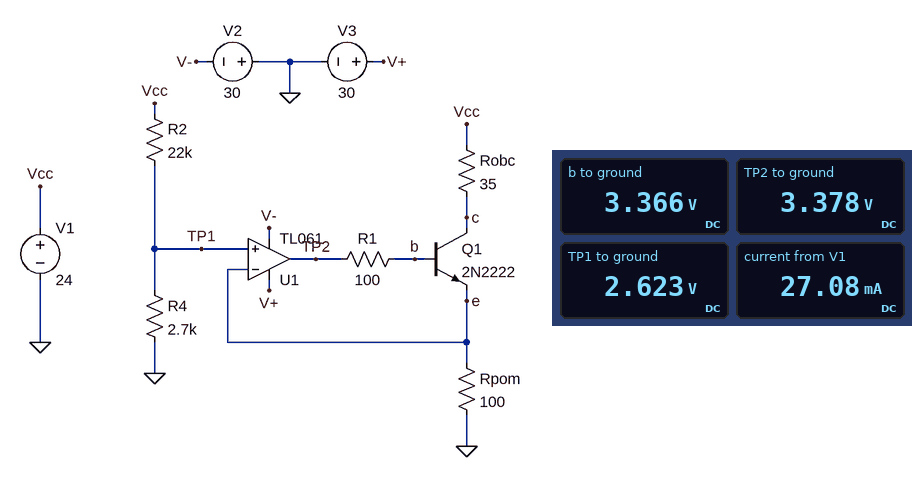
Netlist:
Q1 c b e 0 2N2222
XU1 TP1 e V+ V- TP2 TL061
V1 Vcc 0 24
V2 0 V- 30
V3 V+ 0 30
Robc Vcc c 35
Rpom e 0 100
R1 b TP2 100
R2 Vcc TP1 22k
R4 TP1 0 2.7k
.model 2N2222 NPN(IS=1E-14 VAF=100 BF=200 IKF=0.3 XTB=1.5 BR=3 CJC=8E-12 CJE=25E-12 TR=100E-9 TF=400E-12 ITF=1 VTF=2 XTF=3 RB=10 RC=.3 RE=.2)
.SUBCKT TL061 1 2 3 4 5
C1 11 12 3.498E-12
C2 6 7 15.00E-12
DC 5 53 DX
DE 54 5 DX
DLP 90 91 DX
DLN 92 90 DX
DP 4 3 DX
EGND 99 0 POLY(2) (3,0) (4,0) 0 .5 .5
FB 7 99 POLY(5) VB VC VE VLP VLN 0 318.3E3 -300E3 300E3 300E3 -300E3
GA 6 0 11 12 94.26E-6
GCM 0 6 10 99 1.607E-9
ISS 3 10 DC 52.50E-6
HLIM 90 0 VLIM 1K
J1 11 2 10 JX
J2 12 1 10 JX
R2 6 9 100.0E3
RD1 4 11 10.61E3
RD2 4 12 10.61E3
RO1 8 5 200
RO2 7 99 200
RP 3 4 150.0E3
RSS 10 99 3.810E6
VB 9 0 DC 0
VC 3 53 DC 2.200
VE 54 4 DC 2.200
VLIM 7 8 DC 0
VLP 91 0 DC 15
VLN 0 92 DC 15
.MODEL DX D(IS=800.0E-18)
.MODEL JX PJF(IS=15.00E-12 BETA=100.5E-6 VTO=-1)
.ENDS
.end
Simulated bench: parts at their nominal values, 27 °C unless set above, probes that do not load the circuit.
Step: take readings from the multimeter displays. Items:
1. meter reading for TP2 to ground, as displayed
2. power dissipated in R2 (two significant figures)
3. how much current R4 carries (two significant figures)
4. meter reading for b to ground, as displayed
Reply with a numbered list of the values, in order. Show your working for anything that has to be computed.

1. 3.378 V
2. (24 V - 2.623 V)^2 / 22 kΩ = 21 mW
3. (2.623 V) / 2.7 kΩ = 970 µA
4. 3.366 V
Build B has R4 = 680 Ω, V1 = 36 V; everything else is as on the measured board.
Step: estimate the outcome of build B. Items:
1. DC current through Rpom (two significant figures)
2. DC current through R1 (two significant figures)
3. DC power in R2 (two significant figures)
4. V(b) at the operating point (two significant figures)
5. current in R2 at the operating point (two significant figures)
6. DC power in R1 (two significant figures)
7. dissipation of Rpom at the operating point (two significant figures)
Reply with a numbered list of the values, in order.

1. 11 mA
2. 41 µA
3. 55 mW
4. 1.8 V
5. 1.6 mA
6. 170 nW
7. 12 mW
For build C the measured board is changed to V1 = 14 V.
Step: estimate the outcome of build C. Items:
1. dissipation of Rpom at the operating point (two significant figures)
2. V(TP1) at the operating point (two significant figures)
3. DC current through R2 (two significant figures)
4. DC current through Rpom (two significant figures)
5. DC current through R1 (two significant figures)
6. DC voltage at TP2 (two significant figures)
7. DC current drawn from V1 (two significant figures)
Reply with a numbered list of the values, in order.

1. 23 mW
2. 1.5 V
3. 570 µA
4. 15 mA
5. 72 µA
6. 2.3 V
7. 16 mA
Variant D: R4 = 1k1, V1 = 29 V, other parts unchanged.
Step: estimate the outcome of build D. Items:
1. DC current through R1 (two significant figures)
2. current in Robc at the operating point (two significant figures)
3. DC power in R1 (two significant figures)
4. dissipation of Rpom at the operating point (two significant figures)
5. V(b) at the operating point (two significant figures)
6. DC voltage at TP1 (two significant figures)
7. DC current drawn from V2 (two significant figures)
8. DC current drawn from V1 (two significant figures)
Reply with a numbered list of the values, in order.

1. 56 µA
2. 14 mA
3. 320 nW
4. 19 mW
5. 2.1 V
6. 1.4 V
7. 450 µA
8. 15 mA
